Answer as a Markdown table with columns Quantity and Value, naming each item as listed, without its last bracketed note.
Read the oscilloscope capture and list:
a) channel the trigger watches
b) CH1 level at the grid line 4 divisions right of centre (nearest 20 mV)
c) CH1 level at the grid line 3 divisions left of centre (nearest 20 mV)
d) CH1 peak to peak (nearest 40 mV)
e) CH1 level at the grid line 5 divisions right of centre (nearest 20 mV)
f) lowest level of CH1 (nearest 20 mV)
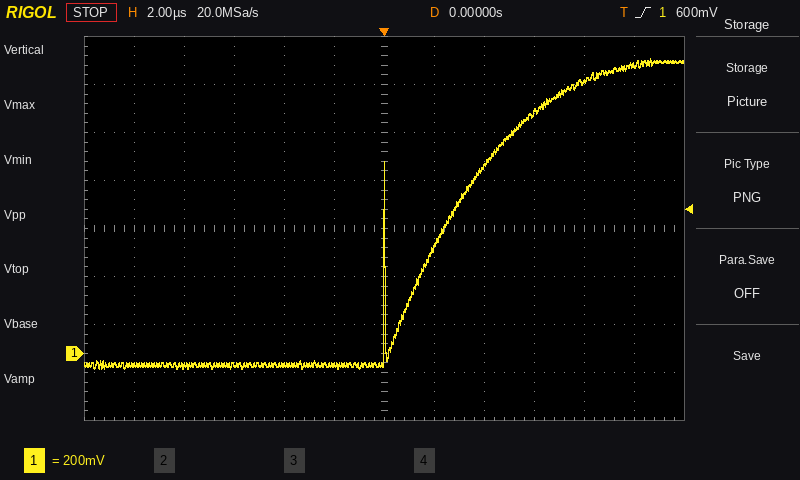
| Quantity | Value |
|---|---|
| channel the trigger watches | CH1 |
| CH1 level at the grid line 4 divisions right of centre | 1.14 V |
| CH1 level at the grid line 3 divisions left of centre | -40 mV |
| CH1 peak to peak | 1.28 V |
| CH1 level at the grid line 5 divisions right of centre | 1.20 V |
| lowest level of CH1 | -60 mV |
